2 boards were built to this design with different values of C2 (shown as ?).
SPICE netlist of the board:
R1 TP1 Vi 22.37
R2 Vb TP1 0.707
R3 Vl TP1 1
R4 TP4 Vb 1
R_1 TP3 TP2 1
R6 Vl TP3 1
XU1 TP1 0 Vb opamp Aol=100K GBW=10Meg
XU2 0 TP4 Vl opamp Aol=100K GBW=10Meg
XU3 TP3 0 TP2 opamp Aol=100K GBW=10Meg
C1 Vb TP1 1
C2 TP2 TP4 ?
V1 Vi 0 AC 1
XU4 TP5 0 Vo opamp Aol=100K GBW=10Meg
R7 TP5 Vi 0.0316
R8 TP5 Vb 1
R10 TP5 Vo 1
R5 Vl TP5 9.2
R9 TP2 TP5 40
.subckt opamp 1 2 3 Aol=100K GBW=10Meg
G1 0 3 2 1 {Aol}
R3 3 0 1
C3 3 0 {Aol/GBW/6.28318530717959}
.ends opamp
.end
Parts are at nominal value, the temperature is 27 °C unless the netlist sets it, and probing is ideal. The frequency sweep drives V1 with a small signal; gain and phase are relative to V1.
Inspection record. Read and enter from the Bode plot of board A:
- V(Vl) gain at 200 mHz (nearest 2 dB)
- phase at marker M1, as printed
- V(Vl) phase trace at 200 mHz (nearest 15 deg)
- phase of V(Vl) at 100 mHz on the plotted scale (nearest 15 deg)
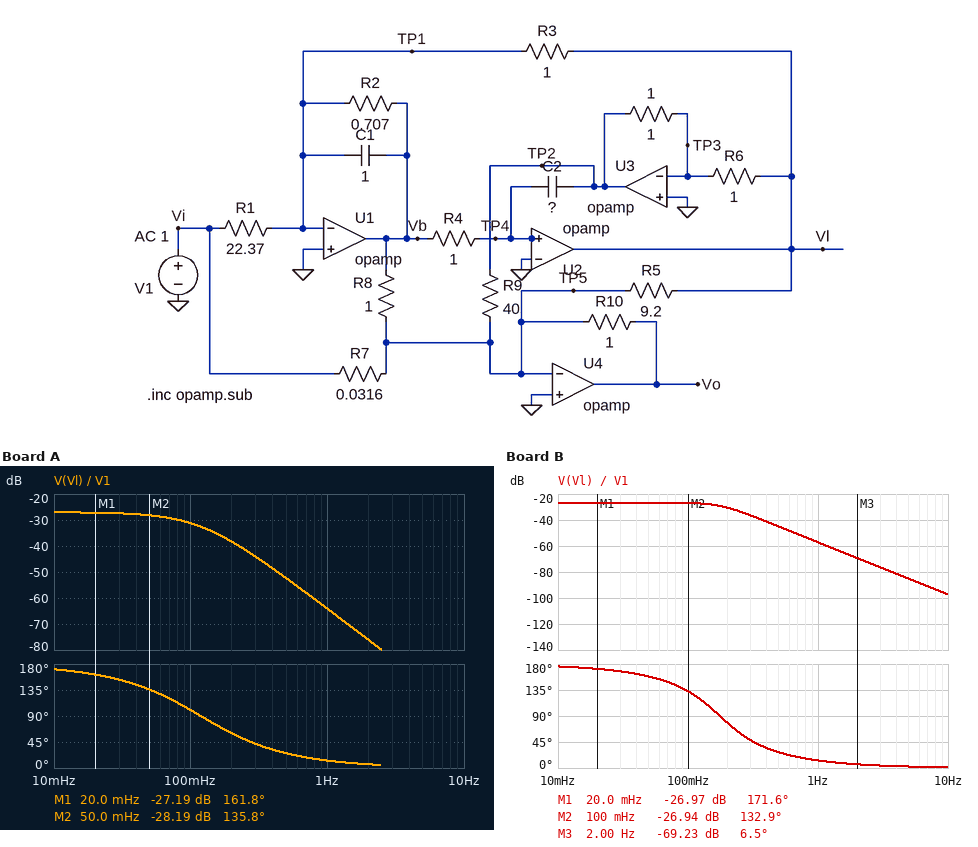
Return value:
-38 dB
161.8 deg
60 deg
105 deg
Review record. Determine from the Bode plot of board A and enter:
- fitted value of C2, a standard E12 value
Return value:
1.8 F
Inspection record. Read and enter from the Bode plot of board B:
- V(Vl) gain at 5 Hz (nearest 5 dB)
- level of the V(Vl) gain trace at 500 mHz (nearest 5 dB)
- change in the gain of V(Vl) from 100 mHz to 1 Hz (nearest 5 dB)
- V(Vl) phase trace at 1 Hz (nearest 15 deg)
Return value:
-85 dB
-45 dB
-30 dB
15 deg
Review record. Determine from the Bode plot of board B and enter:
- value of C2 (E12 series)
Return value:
820 mF
